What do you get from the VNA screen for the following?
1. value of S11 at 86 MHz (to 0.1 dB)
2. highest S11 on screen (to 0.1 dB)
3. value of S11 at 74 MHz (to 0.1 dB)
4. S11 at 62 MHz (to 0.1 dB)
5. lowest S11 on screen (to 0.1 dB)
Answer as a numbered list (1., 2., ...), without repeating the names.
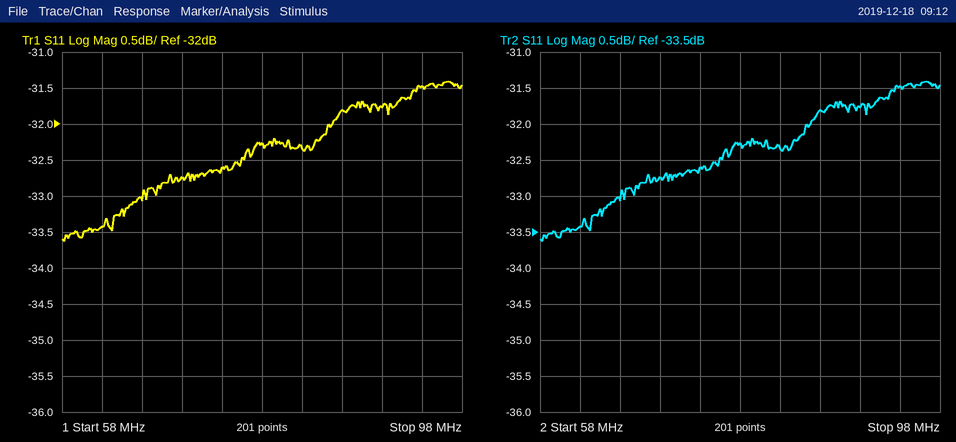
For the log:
1. -31.8 dB
2. -31.4 dB
3. -32.6 dB
4. -33.4 dB
5. -33.6 dB
